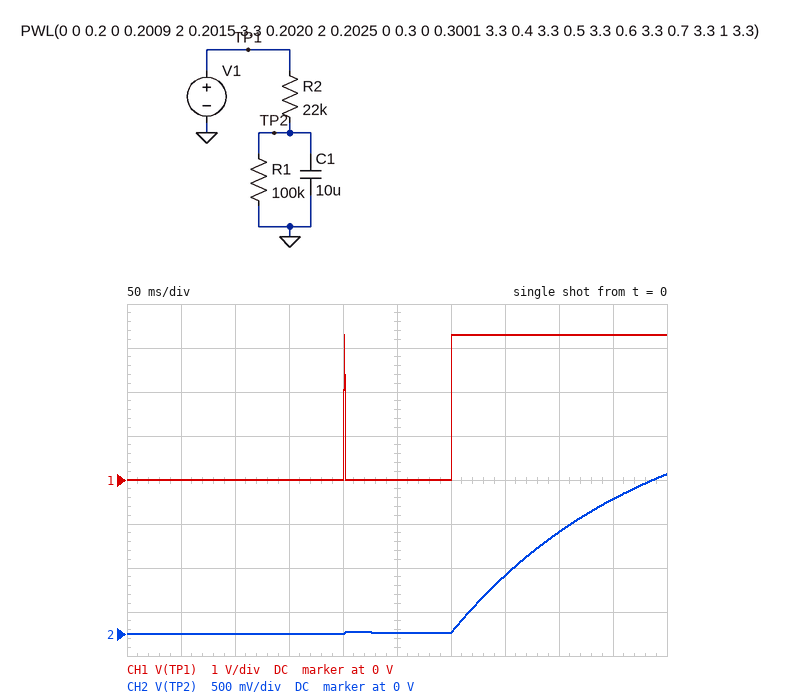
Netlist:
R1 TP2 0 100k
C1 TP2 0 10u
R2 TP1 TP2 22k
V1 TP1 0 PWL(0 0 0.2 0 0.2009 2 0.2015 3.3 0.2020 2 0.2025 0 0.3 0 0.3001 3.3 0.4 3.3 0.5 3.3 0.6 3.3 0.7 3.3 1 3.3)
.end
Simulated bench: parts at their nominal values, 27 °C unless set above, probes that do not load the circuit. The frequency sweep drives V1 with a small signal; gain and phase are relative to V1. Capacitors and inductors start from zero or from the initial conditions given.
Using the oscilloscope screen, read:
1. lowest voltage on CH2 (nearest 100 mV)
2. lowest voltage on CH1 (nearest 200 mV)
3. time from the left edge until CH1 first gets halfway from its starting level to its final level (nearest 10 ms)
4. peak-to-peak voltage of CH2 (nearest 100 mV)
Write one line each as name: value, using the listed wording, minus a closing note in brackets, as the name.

lowest voltage on CH2: 0 V
lowest voltage on CH1: 0 V
time from the left edge until CH1 first gets halfway from its starting level to its final level: 200 ms
peak-to-peak voltage of CH2: 1.8 V
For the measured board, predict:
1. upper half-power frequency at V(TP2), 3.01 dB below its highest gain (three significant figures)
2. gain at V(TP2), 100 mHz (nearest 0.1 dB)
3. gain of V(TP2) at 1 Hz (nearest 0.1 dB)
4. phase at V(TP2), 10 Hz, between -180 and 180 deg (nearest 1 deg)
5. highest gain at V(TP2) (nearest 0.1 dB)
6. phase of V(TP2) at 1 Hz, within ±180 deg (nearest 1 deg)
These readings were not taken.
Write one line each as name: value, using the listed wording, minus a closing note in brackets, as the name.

upper half-power frequency at V(TP2), 3.01 dB below its highest gain: 883 mHz
gain at V(TP2), 100 mHz: -1.8 dB
gain of V(TP2) at 1 Hz: -5.3 dB
phase at V(TP2), 10 Hz, between -180 and 180 deg: -85 deg
highest gain at V(TP2): -1.7 dB
phase of V(TP2) at 1 Hz, within ±180 deg: -49 deg
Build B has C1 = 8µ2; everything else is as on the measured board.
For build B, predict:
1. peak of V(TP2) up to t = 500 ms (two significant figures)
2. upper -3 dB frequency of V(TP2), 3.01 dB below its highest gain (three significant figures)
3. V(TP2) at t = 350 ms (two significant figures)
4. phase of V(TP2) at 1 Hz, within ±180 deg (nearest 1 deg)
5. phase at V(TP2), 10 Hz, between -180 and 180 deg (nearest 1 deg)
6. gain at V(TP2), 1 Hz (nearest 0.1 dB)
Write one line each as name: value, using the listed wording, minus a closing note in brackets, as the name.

peak of V(TP2) up to t = 500 ms: 2.0 V
upper -3 dB frequency of V(TP2), 3.01 dB below its highest gain: 1.08 Hz
V(TP2) at t = 350 ms: 780 mV
phase of V(TP2) at 1 Hz, within ±180 deg: -43 deg
phase at V(TP2), 10 Hz, between -180 and 180 deg: -84 deg
gain at V(TP2), 1 Hz: -4.4 dB
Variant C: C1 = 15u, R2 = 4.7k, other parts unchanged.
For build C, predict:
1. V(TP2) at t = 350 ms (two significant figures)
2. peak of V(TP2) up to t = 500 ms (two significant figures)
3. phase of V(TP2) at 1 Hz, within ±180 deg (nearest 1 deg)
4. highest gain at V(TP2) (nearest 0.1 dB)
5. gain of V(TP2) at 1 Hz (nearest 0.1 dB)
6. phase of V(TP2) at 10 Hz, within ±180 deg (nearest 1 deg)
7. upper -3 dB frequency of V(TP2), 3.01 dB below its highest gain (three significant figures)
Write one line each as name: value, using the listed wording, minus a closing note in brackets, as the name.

V(TP2) at t = 350 ms: 1.7 V
peak of V(TP2) up to t = 500 ms: 3.0 V
phase of V(TP2) at 1 Hz, within ±180 deg: -23 deg
highest gain at V(TP2): -0.4 dB
gain of V(TP2) at 1 Hz: -1.1 dB
phase of V(TP2) at 10 Hz, within ±180 deg: -77 deg
upper -3 dB frequency of V(TP2), 3.01 dB below its highest gain: 2.36 Hz
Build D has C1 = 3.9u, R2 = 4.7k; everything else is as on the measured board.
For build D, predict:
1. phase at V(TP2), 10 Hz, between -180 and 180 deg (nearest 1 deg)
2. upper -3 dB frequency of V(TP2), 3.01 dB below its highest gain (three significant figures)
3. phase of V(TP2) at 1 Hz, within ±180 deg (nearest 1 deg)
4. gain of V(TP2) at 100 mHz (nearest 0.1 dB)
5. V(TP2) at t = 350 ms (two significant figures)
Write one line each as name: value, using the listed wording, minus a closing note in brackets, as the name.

phase at V(TP2), 10 Hz, between -180 and 180 deg: -48 deg
upper -3 dB frequency of V(TP2), 3.01 dB below its highest gain: 9.09 Hz
phase of V(TP2) at 1 Hz, within ±180 deg: -6 deg
gain of V(TP2) at 100 mHz: -0.4 dB
V(TP2) at t = 350 ms: 3.0 V
